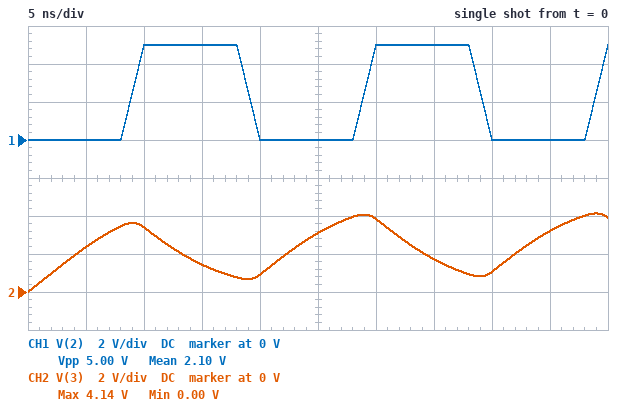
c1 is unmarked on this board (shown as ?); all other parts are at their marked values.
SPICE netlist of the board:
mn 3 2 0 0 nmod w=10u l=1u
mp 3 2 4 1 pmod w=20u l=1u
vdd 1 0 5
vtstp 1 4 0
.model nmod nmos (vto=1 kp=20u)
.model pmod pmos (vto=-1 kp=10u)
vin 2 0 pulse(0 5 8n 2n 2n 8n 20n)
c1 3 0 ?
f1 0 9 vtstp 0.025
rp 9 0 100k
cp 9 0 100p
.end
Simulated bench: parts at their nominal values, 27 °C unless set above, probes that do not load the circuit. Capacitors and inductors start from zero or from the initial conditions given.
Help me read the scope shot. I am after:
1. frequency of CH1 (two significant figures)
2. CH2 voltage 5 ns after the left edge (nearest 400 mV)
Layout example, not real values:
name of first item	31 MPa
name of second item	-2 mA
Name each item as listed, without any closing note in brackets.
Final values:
frequency of CH1	50 MHz
CH2 voltage 5 ns after the left edge	2.4 V
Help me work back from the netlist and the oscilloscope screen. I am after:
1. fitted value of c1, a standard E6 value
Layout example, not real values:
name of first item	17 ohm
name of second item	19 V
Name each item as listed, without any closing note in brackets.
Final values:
fitted value of c1, a standard E6 value	3.3 pF
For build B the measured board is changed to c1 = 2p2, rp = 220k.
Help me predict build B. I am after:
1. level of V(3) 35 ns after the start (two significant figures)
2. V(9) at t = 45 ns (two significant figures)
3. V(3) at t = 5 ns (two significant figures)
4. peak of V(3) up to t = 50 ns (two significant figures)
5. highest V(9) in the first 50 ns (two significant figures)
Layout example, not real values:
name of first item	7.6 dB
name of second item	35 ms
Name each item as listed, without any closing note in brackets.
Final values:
level of V(3) 35 ns after the start	1.2 V
V(9) at t = 45 ns	6.7 mV
V(3) at t = 5 ns	3.3 V
peak of V(3) up to t = 50 ns	4.6 V
highest V(9) in the first 50 ns	7.2 mV
